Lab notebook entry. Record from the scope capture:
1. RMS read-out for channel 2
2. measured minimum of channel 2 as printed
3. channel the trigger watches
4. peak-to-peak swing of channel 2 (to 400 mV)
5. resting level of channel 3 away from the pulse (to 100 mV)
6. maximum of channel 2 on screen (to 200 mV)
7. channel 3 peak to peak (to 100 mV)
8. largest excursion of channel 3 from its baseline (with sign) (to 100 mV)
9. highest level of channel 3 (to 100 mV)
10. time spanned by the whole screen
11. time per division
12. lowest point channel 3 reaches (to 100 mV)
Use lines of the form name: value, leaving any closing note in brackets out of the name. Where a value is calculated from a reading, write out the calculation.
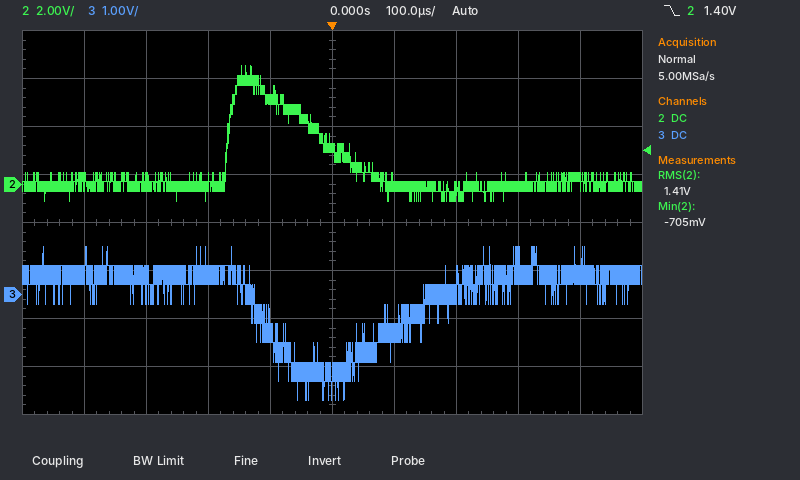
RMS read-out for channel 2: 1.41 V
measured minimum of channel 2 as printed: -705 mV
channel the trigger watches: channel 2
peak-to-peak swing of channel 2: 5.6 V
resting level of channel 3 away from the pulse: 400 mV
maximum of channel 2 on screen: 5.0 V
channel 3 peak to peak: 1.0 V − (-2.2 V) = 3.2 V
largest excursion of channel 3 from its baseline (with sign): -2.2 V − (400 mV) = -2.6 V
highest level of channel 3: 1.0 V
time spanned by the whole screen: 1 ms
time per division: 100 µs
lowest point channel 3 reaches: -2.2 V
